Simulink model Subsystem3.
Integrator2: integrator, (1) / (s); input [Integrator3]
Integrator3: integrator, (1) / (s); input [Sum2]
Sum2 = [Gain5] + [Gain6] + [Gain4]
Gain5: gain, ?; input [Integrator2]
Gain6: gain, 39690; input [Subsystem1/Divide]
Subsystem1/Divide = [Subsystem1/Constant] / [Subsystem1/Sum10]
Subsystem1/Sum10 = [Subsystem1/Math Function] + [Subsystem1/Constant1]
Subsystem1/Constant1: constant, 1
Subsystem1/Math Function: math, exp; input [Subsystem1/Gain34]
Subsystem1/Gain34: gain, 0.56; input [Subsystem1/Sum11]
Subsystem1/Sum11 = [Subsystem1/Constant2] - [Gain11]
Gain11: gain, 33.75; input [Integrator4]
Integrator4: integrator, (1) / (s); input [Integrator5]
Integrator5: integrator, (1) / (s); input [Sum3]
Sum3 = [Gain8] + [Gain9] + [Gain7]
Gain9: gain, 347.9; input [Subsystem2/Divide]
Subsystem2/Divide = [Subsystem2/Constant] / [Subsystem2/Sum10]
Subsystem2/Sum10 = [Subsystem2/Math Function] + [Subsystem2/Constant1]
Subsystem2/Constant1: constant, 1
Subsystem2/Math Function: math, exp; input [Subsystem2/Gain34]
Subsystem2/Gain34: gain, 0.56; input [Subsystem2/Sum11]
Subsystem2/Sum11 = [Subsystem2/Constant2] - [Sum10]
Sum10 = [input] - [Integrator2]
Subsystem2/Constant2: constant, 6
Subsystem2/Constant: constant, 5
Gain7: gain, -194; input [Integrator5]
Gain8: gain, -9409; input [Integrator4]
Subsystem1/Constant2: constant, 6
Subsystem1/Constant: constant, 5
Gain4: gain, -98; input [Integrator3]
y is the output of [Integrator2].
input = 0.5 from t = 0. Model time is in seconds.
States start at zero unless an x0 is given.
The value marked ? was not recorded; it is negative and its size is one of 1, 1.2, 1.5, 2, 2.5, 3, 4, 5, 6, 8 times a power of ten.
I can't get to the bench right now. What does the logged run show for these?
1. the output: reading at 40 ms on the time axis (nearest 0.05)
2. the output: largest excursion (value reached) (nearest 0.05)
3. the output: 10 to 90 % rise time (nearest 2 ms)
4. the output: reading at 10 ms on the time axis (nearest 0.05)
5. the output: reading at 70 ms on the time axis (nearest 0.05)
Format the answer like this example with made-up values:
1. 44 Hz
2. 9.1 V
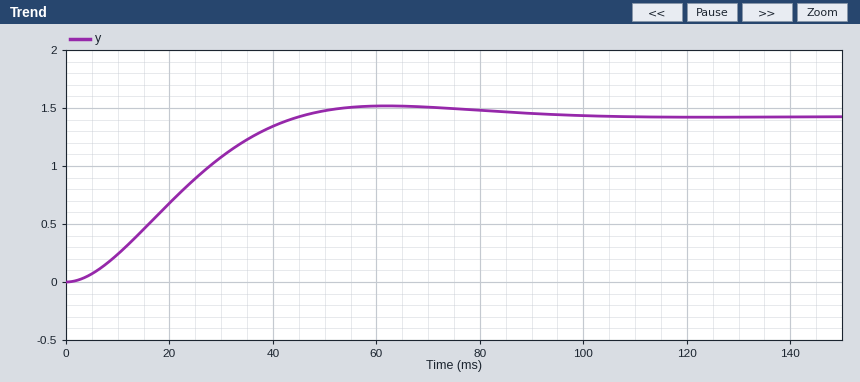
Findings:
1. 1.35
2. 1.50
3. 30 ms
4. 0.25
5. 1.50
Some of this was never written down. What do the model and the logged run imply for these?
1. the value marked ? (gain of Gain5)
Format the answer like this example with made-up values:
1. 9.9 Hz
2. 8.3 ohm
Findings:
1. -5000
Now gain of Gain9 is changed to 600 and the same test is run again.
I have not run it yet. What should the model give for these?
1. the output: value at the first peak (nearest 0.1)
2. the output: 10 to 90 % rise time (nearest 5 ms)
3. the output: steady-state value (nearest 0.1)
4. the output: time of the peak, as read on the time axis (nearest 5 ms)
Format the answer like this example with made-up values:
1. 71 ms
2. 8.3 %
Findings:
1. 1.6
2. 30 ms
3. 1.5
4. 60 ms
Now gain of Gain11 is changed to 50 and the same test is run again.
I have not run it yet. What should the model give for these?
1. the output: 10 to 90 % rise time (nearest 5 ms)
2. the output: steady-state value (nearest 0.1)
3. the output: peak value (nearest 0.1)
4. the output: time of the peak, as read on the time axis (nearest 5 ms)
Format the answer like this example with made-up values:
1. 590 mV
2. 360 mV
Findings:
1. 30 ms
2. 1.5
3. 1.6
4. 60 ms
